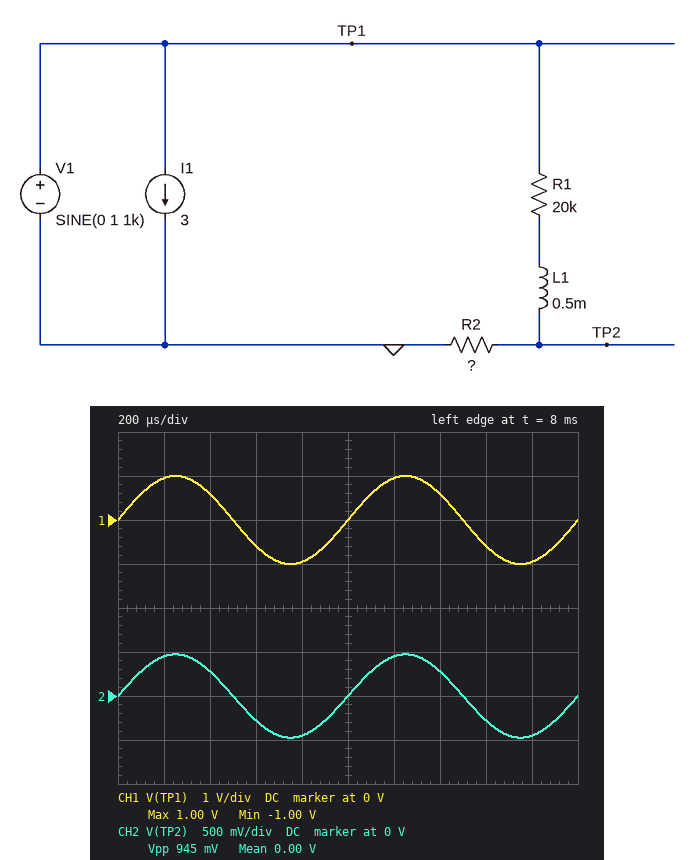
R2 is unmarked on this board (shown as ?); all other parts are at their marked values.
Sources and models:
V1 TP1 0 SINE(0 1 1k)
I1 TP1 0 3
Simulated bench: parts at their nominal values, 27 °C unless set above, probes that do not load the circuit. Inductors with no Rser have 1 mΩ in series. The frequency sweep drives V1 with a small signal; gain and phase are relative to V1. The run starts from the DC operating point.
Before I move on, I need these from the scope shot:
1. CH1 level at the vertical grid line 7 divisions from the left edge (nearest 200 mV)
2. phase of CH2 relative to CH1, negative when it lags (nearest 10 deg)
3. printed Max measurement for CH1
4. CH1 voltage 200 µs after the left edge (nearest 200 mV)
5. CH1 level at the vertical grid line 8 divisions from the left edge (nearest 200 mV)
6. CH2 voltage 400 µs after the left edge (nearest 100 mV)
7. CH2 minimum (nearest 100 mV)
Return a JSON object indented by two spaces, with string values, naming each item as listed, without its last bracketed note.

{
  "CH1 level at the vertical grid line 7 divisions from the left edge": "600 mV",
  "phase of CH2 relative to CH1, negative when it lags": "0 deg",
  "printed Max measurement for CH1": "1.00 V",
  "CH1 voltage 200 µs after the left edge": "1.0 V",
  "CH1 level at the vertical grid line 8 divisions from the left edge": "-600 mV",
  "CH2 voltage 400 µs after the left edge": "300 mV",
  "CH2 minimum": "-500 mV"
}
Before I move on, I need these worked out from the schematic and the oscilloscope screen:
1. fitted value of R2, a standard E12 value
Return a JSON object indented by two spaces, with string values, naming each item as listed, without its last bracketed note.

{
  "fitted value of R2, a standard E12 value": "18 kΩ"
}
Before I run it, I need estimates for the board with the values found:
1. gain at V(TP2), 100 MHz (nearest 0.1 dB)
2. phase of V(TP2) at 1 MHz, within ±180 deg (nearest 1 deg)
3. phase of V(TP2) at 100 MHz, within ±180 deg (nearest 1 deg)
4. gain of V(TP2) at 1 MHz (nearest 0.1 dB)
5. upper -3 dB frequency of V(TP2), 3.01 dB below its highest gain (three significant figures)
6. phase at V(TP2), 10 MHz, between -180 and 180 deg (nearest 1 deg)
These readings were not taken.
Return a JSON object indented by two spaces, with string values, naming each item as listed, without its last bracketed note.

{
  "gain at V(TP2), 100 MHz": "-24.9 dB",
  "phase of V(TP2) at 1 MHz, within ±180 deg": "-5 deg",
  "phase of V(TP2) at 100 MHz, within ±180 deg": "-83 deg",
  "gain of V(TP2) at 1 MHz": "-6.5 dB",
  "upper -3 dB frequency of V(TP2), 3.01 dB below its highest gain": "12.1 MHz",
  "phase at V(TP2), 10 MHz, between -180 and 180 deg": "-40 deg"
}
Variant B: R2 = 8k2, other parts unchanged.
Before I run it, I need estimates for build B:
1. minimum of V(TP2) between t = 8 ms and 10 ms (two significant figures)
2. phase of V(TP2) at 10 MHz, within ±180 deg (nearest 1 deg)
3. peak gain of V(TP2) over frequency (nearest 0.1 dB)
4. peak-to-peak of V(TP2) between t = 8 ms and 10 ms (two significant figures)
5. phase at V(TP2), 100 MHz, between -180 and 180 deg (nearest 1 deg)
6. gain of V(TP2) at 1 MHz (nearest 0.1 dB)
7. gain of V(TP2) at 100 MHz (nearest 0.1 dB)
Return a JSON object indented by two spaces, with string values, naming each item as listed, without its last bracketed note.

{
  "minimum of V(TP2) between t = 8 ms and 10 ms": "-290 mV",
  "phase of V(TP2) at 10 MHz, within ±180 deg": "-48 deg",
  "peak gain of V(TP2) over frequency": "-10.7 dB",
  "peak-to-peak of V(TP2) between t = 8 ms and 10 ms": "580 mV",
  "phase at V(TP2), 100 MHz, between -180 and 180 deg": "-85 deg",
  "gain of V(TP2) at 1 MHz": "-10.8 dB",
  "gain of V(TP2) at 100 MHz": "-31.7 dB"
}
